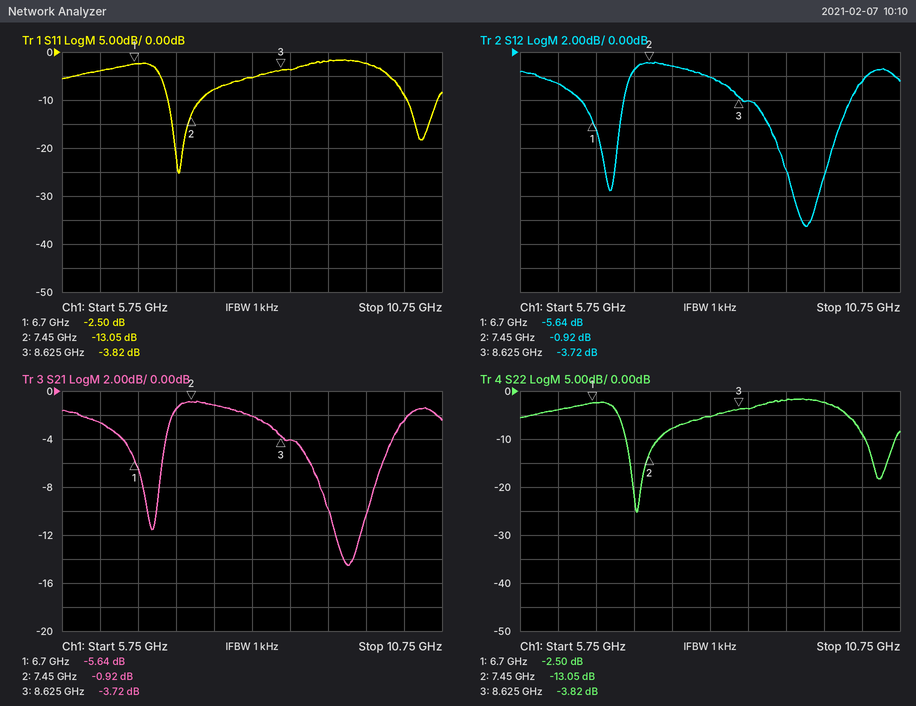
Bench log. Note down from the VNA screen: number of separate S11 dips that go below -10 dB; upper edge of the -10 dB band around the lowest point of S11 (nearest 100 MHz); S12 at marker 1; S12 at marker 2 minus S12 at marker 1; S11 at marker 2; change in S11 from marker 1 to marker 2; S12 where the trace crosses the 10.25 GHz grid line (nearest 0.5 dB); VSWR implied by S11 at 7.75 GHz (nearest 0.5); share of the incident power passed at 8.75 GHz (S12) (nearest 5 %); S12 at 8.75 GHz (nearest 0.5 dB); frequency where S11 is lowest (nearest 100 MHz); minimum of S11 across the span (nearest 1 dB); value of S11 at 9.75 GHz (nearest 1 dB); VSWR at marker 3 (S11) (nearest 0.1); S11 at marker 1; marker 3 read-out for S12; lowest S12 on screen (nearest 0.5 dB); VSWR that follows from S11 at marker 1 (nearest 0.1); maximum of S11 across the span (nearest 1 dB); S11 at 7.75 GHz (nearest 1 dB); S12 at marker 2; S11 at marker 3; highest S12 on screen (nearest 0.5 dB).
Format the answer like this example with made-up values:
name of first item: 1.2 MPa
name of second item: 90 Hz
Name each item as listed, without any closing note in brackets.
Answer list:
number of separate S11 dips that go below -10 dB: 2
upper edge of the -10 dB band around the lowest point of S11: 7.6 GHz
S12 at marker 1: -5.64 dB
S12 at marker 2 minus S12 at marker 1: 4.72 dB
S11 at marker 2: -13.05 dB
change in S11 from marker 1 to marker 2: -10.55 dB
S12 where the trace crosses the 10.25 GHz grid line: -2.5 dB
VSWR implied by S11 at 7.75 GHz: 2.5
share of the incident power passed at 8.75 GHz (S12): 40 %
S12 at 8.75 GHz: -4.0 dB
frequency where S11 is lowest: 7.3 GHz
minimum of S11 across the span: -25 dB
value of S11 at 9.75 GHz: -2 dB
VSWR at marker 3 (S11): 4.6
S11 at marker 1: -2.50 dB
marker 3 read-out for S12: -3.72 dB
lowest S12 on screen: -14.5 dB
VSWR that follows from S11 at marker 1: 7.0
maximum of S11 across the span: -2 dB
S11 at 7.75 GHz: -8 dB
S12 at marker 2: -0.92 dB
S11 at marker 3: -3.82 dB
highest S12 on screen: -1.0 dB
